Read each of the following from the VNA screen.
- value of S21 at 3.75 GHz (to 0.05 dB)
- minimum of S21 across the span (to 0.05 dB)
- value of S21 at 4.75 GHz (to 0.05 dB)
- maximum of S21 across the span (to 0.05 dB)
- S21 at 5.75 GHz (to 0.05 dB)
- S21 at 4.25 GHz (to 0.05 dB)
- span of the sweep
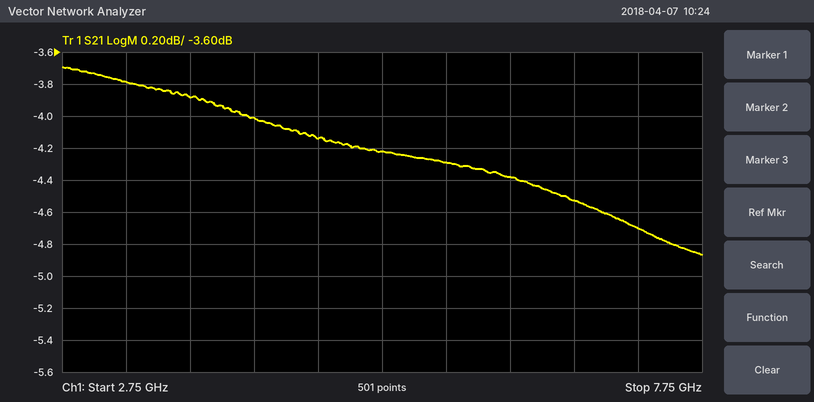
-3.90 dB
-4.85 dB
-4.15 dB
-3.70 dB
-4.30 dB
-4.00 dB
5 GHz
